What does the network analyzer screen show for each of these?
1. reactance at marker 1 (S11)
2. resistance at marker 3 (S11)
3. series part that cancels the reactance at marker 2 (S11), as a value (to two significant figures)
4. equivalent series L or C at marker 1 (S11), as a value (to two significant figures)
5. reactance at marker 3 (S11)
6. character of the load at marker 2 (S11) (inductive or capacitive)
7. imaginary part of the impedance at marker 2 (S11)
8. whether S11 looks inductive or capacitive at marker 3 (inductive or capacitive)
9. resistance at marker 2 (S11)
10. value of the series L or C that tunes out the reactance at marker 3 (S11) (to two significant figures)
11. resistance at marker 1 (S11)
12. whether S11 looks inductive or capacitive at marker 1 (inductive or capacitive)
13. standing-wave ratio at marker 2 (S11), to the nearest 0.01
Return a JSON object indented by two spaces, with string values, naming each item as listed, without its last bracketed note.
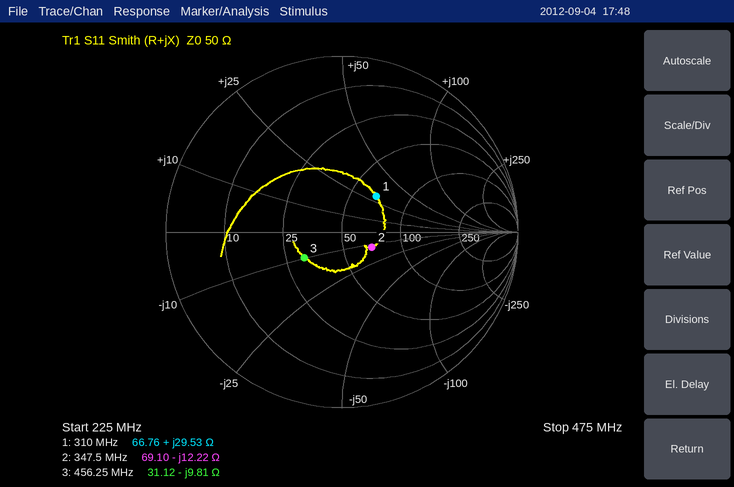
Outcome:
{
  "reactance at marker 1": "+29.53 Ω",
  "resistance at marker 3": "31.12 Ω",
  "series part that cancels the reactance at marker 2 (S11), as a value": "5.6 nH",
  "equivalent series L or C at marker 1 (S11), as a value": "15 nH",
  "reactance at marker 3": "-9.81 Ω",
  "character of the load at marker 2 (S11)": "capacitive",
  "imaginary part of the impedance at marker 2": "-12.22 Ω",
  "whether S11 looks inductive or capacitive at marker 3": "capacitive",
  "resistance at marker 2": "69.10 Ω",
  "value of the series L or C that tunes out the reactance at marker 3 (S11)": "3.4 nH",
  "resistance at marker 1": "66.76 Ω",
  "whether S11 looks inductive or capacitive at marker 1": "inductive",
  "standing-wave ratio at marker 2 (S11), to the nearest 0.01": "1.47"
}
